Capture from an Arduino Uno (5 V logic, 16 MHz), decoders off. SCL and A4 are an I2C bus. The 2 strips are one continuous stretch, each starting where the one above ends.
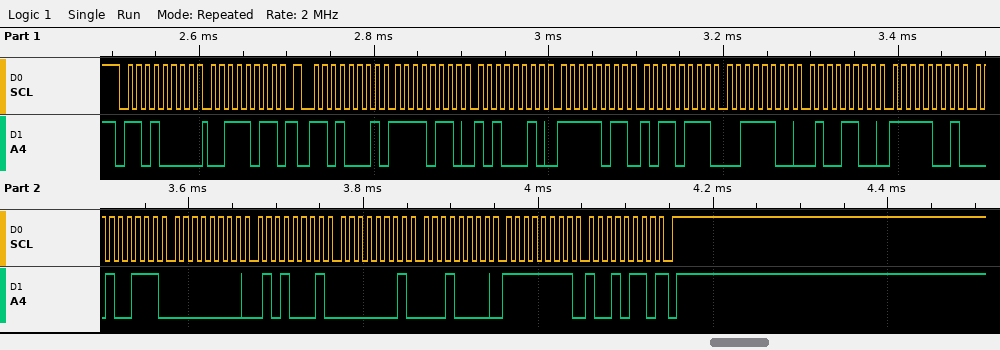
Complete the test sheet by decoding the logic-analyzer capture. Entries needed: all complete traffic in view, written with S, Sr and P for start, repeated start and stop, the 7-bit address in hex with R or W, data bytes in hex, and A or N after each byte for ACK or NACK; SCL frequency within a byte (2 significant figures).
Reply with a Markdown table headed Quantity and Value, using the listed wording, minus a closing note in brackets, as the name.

| Quantity | Value |
|---|---|
| all complete traffic in view, written with S, Sr and P for start, repeated start and stop, the 7-bit address in hex with R or W, data bytes in hex, and A or N after each byte for ACK or NACK | S 68W A 3B A Sr 68R A F6 A A2 A FB A B7 A 3C A 4C A F9 A 27 A 00 A 51 A 01 A 10 A FF A 96 N P |
| SCL frequency within a byte | 100 kHz |
